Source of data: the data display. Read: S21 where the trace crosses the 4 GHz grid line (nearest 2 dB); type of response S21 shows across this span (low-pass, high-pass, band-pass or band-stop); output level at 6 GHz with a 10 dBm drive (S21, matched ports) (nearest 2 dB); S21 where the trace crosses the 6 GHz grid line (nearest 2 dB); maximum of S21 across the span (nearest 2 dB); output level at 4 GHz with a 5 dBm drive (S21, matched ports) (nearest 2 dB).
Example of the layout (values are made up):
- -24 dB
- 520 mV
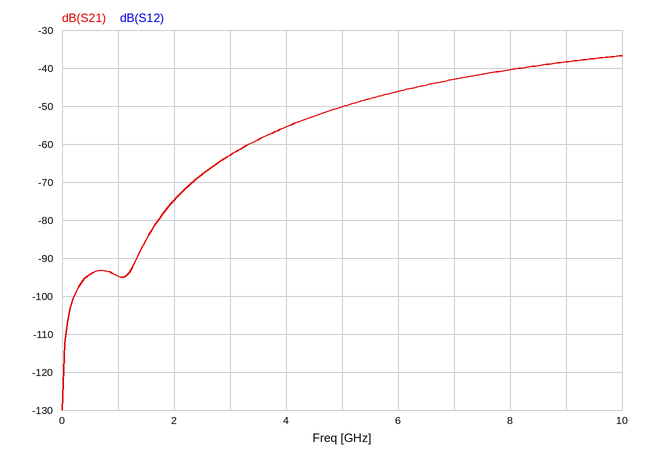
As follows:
- -56 dB
- high-pass
- -36 dBm
- -46 dB
- -36 dB
- -50 dBm
